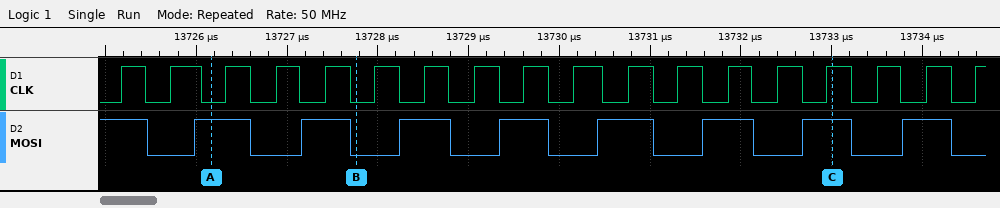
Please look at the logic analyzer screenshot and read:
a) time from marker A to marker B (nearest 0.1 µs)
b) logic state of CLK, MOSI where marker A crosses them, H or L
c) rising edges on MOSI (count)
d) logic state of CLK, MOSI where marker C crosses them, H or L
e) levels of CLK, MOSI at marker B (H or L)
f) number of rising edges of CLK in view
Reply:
1.6 µs
CLK=L, MOSI=H
8
CLK=H, MOSI=H
CLK=L, MOSI=L
18
